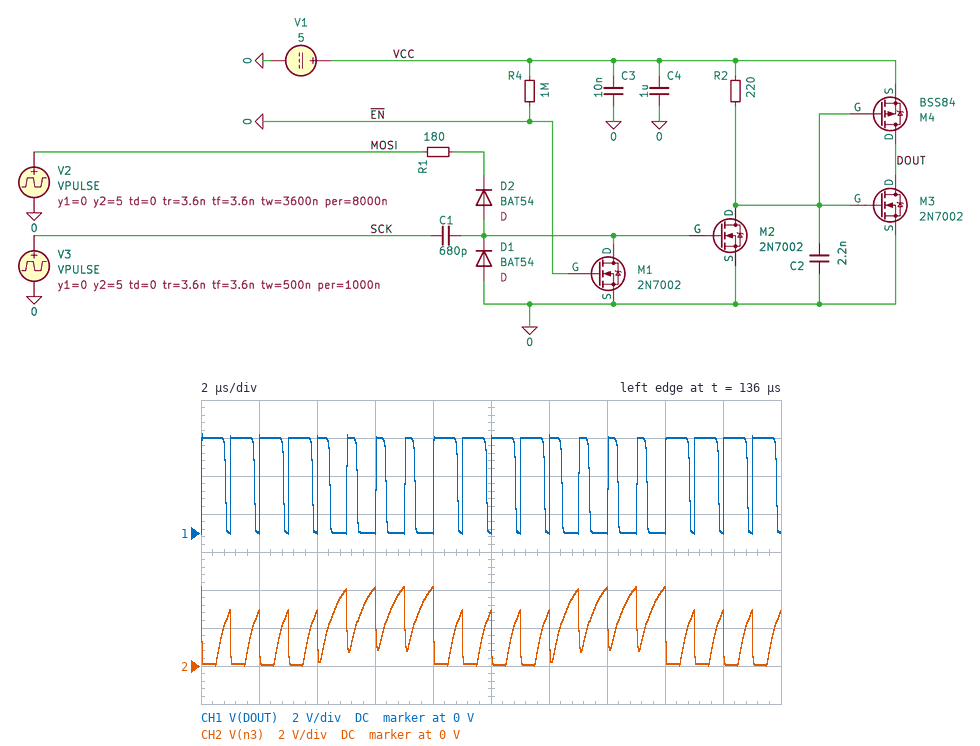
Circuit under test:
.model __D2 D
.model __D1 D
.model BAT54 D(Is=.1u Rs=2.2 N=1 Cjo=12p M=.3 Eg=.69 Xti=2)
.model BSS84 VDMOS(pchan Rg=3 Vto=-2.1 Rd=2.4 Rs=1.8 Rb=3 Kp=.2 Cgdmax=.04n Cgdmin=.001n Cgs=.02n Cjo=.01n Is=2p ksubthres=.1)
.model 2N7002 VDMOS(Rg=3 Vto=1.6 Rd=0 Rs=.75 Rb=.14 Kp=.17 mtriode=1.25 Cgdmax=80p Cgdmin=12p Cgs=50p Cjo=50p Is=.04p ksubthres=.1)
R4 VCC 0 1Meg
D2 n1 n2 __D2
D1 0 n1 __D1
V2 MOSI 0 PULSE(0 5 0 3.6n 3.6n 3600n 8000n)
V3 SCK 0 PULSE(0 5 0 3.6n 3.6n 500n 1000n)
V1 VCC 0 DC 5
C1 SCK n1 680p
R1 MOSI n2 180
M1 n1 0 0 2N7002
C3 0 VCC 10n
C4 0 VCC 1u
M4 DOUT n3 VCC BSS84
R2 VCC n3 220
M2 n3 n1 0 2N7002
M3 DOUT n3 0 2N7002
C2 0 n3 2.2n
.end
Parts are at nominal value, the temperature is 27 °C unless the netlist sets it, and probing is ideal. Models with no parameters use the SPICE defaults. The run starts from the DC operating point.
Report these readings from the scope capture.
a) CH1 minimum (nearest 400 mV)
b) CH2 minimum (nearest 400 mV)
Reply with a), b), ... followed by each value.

a) 0 V
b) 0 V
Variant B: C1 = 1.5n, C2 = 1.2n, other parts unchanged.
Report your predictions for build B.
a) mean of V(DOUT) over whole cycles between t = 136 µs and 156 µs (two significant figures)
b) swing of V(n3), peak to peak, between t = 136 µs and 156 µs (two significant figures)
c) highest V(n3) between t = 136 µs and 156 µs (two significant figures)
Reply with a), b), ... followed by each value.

a) 3.1 V
b) 4.6 V
c) 4.5 V
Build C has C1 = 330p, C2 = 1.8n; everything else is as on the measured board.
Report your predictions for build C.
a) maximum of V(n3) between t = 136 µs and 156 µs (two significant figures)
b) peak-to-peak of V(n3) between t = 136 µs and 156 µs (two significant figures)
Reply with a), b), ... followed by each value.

a) 4.9 V
b) 4.8 V
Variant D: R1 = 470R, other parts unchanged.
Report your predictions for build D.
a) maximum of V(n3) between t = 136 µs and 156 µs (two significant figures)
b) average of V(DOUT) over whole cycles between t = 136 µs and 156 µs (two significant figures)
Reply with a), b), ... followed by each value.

a) 3.6 V
b) 3.7 V
